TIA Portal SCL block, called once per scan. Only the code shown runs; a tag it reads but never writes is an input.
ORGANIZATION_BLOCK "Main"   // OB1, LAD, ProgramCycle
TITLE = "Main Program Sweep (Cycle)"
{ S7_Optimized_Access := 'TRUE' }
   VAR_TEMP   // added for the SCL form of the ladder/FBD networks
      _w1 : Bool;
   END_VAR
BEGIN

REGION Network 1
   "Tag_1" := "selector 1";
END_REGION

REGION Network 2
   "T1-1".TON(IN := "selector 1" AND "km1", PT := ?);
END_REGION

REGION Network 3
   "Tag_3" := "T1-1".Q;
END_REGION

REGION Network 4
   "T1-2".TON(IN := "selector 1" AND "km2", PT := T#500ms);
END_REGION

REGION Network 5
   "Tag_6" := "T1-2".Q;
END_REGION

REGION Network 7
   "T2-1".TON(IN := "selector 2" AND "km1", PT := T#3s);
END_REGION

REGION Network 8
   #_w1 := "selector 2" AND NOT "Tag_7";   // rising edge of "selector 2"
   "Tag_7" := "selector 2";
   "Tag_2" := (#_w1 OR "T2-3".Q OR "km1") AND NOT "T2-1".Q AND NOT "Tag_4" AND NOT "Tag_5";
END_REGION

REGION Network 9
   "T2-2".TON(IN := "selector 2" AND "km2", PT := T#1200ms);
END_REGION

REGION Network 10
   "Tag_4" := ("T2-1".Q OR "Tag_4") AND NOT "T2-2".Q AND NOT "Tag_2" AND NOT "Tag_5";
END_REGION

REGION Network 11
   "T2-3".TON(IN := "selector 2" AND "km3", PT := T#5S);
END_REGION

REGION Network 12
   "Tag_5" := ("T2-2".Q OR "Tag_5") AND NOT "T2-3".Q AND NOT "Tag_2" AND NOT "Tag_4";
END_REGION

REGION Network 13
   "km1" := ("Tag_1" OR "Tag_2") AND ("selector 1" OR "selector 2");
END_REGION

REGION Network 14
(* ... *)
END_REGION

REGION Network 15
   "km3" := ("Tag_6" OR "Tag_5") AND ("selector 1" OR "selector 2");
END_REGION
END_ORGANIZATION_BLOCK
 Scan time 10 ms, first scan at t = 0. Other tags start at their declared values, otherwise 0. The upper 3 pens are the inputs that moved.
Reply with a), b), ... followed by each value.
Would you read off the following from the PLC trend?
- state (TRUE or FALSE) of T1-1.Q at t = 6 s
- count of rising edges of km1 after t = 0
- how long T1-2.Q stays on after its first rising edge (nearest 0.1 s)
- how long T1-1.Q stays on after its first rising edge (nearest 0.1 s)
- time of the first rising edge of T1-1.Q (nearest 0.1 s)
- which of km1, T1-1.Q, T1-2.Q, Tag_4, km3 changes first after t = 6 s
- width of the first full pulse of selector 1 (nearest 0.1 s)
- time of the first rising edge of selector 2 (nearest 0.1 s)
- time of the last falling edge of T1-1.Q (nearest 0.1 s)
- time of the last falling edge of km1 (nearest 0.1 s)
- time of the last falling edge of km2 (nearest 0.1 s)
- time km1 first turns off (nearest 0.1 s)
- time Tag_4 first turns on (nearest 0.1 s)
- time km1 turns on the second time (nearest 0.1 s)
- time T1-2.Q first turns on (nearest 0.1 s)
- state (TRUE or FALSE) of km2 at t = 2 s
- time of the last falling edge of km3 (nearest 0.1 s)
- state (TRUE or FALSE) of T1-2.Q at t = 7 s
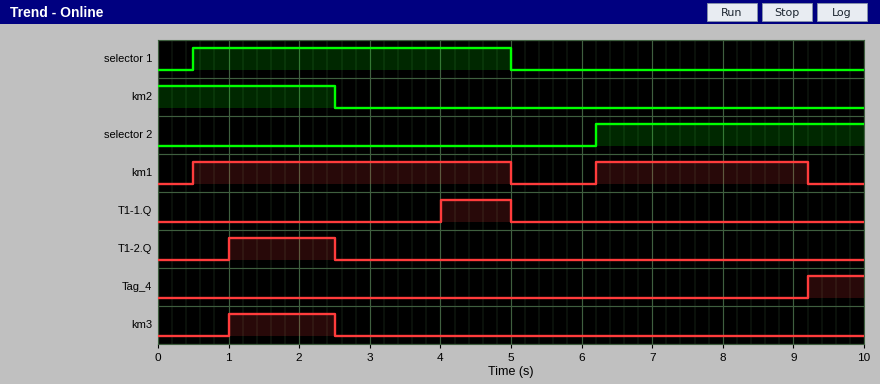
a) FALSE
b) 2
c) 1.5 s
d) 1.0 s
e) 4.0 s
f) km1
g) 4.5 s
h) 6.2 s
i) 5.0 s
j) 9.2 s
k) 2.5 s
l) 5.0 s
m) 9.2 s
n) 6.2 s
o) 1.0 s
p) TRUE
q) 2.5 s
r) FALSE
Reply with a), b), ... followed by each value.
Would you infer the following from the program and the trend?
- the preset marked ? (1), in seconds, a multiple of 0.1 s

a) 3.5 s
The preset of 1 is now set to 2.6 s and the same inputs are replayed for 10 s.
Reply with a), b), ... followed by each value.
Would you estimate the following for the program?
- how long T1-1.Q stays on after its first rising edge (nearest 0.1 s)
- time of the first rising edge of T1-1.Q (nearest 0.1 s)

a) 1.9 s
b) 3.1 s
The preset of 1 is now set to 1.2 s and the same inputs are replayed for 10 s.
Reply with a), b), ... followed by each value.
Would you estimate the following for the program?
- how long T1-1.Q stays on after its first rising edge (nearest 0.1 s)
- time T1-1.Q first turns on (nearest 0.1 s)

a) 3.3 s
b) 1.7 s
